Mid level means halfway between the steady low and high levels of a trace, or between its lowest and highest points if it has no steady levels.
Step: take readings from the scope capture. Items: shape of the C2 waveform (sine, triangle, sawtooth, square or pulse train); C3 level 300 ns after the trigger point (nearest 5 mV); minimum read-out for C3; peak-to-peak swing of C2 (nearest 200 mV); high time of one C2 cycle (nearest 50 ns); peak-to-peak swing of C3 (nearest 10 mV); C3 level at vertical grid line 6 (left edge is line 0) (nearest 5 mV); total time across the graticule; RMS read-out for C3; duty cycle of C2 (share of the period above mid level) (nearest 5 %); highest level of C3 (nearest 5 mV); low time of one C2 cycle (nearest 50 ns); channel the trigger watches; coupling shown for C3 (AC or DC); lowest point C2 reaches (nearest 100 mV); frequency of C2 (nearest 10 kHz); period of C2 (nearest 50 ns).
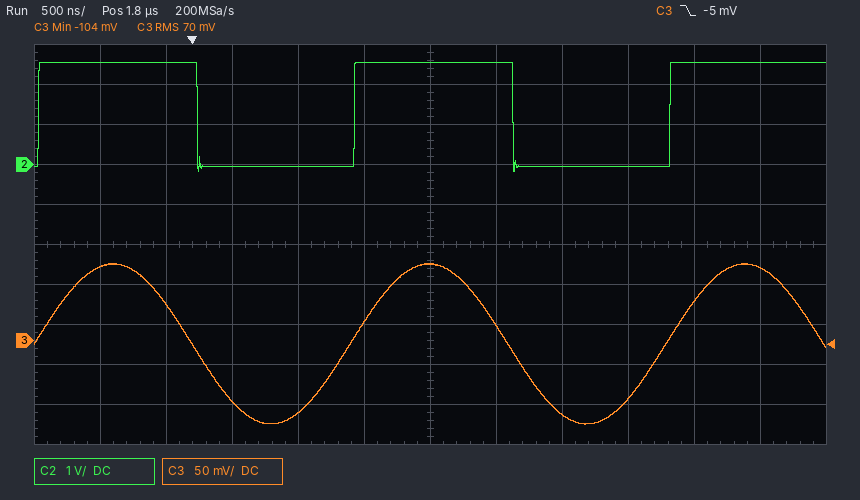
square
-75 mV
-104 mV
2.8 V
1.20 µs
200 mV
95 mV
6 µs
70 mV
50 %
95 mV
1.20 µs
C3
DC
-200 mV
420 kHz
2.40 µs
